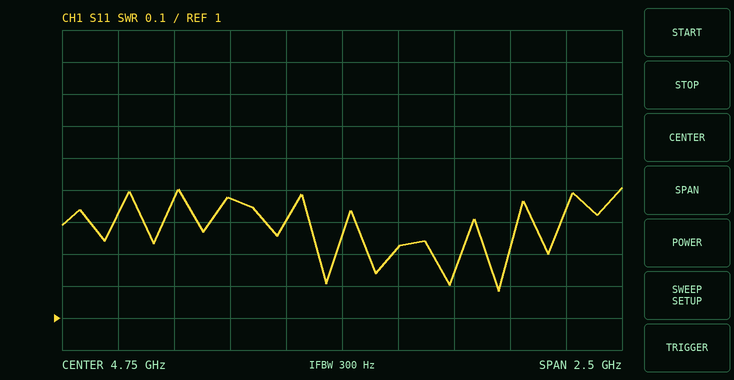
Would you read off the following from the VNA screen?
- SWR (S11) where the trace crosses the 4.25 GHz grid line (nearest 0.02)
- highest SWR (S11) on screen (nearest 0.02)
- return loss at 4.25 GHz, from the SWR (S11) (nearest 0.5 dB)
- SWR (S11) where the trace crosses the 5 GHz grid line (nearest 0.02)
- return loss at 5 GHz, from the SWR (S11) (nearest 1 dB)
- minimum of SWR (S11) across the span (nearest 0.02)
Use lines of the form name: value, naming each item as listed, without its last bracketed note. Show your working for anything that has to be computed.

SWR (S11) where the trace crosses the 4.25 GHz grid line: 1.38
highest SWR (S11) on screen: 1.40
return loss at 4.25 GHz, from the SWR (S11): −20 log10((1.38 − 1)/(1.38 + 1)) ≈ 15.9 dB, so 16.0 dB to the nearest 0.5 dB
SWR (S11) where the trace crosses the 5 GHz grid line: 1.22
return loss at 5 GHz, from the SWR (S11): −20 log10((1.22 − 1)/(1.22 + 1)) ≈ 20 dB
minimum of SWR (S11) across the span: 1.08
